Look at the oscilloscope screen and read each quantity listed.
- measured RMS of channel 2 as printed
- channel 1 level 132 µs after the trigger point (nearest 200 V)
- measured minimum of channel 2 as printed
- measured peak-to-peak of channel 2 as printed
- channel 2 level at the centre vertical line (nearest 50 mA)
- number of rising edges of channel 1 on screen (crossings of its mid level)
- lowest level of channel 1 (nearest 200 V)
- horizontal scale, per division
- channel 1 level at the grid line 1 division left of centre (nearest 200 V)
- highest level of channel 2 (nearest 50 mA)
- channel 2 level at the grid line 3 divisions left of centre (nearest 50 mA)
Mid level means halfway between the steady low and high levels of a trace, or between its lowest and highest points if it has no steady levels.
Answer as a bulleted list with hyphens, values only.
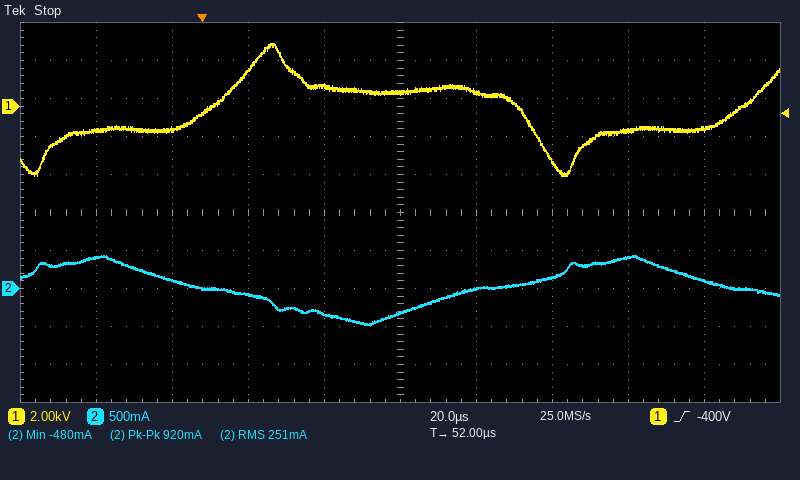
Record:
- 251 mA
- -1.2 kV
- -480 mA
- 920 mA
- -300 mA
- 2
- -3.6 kV
- 20 µs
- 1.0 kV
- 450 mA
- 100 mA
